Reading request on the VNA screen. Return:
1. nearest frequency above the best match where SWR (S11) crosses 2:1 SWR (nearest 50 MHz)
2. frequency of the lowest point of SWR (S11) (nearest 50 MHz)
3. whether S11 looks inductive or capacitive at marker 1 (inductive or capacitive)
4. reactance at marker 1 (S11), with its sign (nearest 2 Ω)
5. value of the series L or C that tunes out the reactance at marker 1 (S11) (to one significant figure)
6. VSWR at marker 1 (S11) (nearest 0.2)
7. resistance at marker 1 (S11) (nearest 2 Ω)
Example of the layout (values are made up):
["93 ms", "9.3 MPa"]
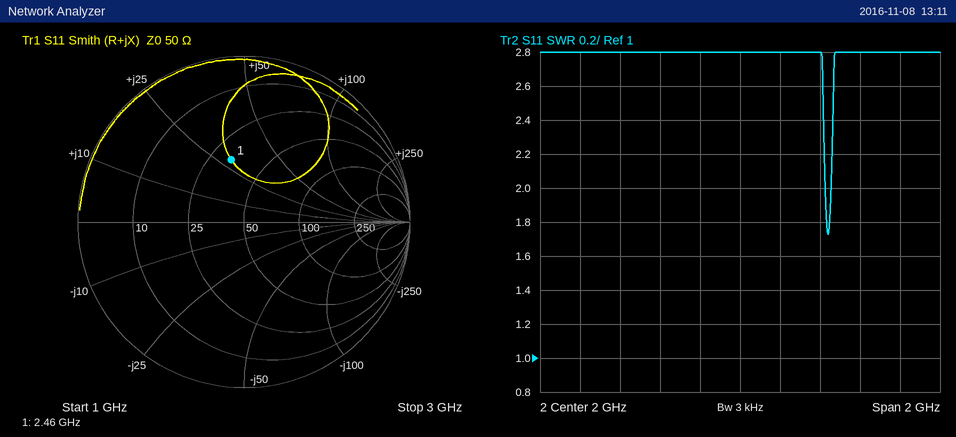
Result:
["2.45 GHz", "2.45 GHz", "inductive", "+28 Ω", "2 pF", "2.2", "32 Ω"]
